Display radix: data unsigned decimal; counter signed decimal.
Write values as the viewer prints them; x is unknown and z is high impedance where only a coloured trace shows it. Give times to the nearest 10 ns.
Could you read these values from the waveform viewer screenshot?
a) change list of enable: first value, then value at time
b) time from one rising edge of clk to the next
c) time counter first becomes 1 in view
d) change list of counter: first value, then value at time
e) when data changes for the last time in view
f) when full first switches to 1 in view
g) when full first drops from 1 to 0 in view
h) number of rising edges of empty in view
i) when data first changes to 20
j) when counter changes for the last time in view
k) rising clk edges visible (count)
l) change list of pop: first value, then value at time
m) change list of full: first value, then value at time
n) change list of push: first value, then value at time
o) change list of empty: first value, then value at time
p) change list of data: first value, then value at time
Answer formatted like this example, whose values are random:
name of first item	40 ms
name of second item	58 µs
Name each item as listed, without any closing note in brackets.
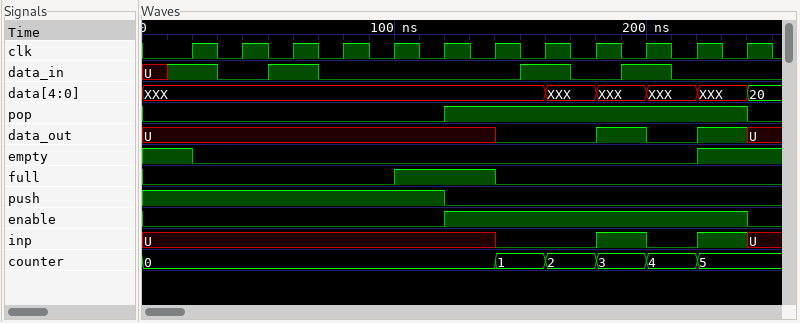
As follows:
change list of enable: first value, then value at time	0, 1 at 120 ns, 0 at 240 ns
time from one rising edge of clk to the next	20 ns
time counter first becomes 1 in view	140 ns
change list of counter: first value, then value at time	0, 1 at 140 ns, 2 at 160 ns, 3 at 180 ns, 4 at 200 ns, 5 at 220 ns
when data changes for the last time in view	240 ns
when full first switches to 1 in view	100 ns
when full first drops from 1 to 0 in view	140 ns
number of rising edges of empty in view	1
when data first changes to 20	240 ns
when counter changes for the last time in view	220 ns
rising clk edges visible	12
change list of pop: first value, then value at time	0, 1 at 120 ns, 0 at 240 ns
change list of full: first value, then value at time	0, 1 at 100 ns, 0 at 140 ns
change list of push: first value, then value at time	1, 0 at 120 ns
change list of empty: first value, then value at time	1, 0 at 20 ns, 1 at 220 ns
change list of data: first value, then value at time	XXX, XXX at 160 ns, XXX at 180 ns, XXX at 200 ns, XXX at 220 ns, 20 at 240 ns
